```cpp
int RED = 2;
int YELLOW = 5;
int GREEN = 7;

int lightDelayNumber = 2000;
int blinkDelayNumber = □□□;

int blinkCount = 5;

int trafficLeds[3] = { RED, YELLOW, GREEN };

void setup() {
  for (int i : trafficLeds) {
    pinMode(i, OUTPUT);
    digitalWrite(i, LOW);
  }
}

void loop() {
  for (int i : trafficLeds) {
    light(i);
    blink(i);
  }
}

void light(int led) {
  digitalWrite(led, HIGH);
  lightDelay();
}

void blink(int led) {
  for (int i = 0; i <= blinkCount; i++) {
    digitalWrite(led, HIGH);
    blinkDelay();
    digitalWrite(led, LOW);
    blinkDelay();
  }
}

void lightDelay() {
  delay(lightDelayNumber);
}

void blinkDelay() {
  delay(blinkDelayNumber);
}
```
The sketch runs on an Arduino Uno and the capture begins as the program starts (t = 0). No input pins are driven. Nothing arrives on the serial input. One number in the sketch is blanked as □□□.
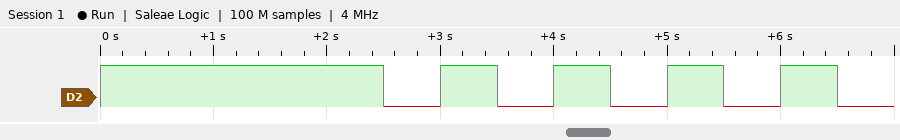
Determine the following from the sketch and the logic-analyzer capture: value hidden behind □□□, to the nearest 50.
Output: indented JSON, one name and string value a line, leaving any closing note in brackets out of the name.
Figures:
{
  "value hidden behind □□□, to the nearest 50": "500"
}
